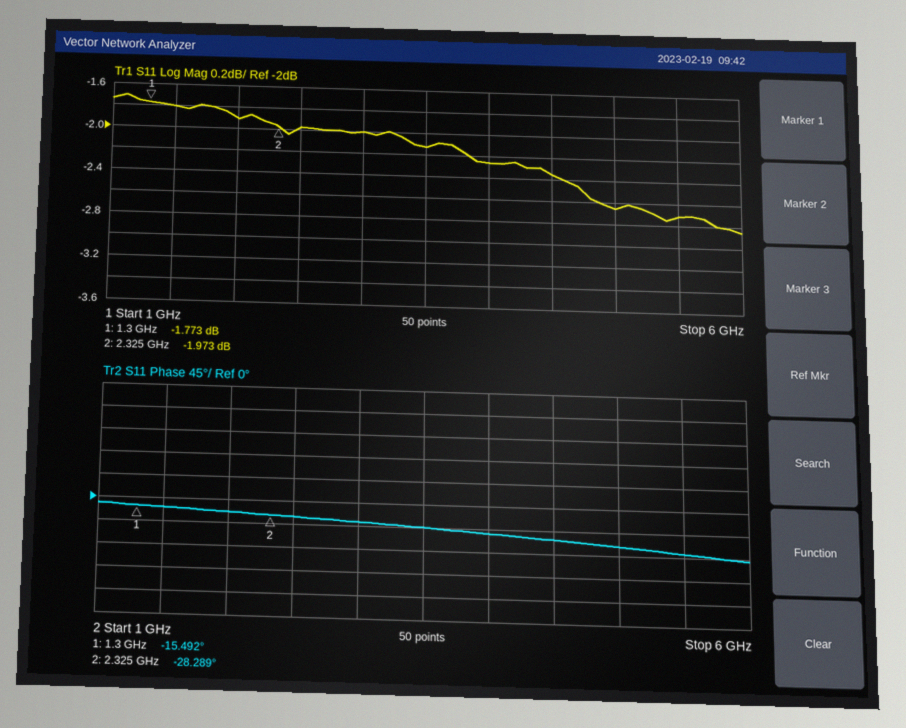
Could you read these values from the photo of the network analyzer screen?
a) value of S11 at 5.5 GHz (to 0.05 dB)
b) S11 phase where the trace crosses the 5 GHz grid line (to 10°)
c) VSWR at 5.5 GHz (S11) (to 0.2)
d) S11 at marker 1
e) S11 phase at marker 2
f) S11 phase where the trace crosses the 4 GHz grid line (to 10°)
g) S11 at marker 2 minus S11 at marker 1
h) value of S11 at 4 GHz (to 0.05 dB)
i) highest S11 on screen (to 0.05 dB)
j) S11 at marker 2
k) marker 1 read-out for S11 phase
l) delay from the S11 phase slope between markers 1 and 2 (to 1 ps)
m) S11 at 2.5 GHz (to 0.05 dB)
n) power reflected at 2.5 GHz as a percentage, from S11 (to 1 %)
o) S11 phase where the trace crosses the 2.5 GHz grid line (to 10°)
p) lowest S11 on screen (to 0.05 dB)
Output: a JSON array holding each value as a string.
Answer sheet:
["-2.70 dB", "-70°", "6.4", "-1.773 dB", "-28.289°", "-50°", "-0.200 dB", "-2.25 dB", "-1.70 dB", "-1.973 dB", "-15.492°", "35 ps", "-2.00 dB", "63 %", "-30°", "-2.85 dB"]
